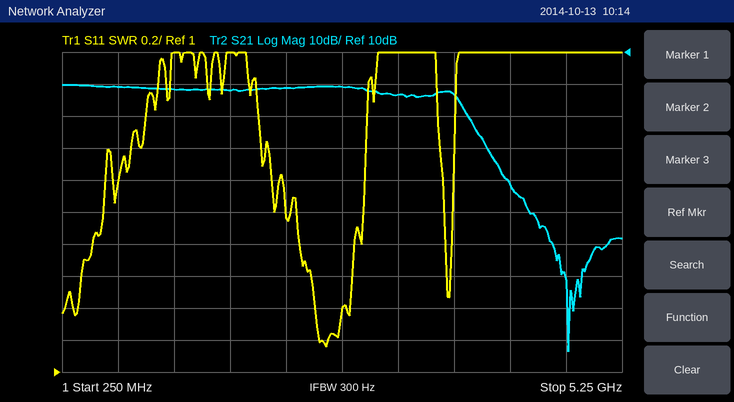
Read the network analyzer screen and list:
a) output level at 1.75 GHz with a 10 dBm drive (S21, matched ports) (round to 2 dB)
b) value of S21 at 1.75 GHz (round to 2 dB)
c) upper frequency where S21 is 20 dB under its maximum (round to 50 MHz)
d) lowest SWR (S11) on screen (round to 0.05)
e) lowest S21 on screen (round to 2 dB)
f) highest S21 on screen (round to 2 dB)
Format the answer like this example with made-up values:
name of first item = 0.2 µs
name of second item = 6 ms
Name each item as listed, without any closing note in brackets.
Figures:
output level at 1.75 GHz with a 10 dBm drive (S21, matched ports) = 8 dBm
value of S21 at 1.75 GHz = -2 dB
upper frequency where S21 is 20 dB under its maximum = 4.05 GHz
lowest SWR (S11) on screen = 1.15
lowest S21 on screen = -84 dB
highest S21 on screen = 0 dB
